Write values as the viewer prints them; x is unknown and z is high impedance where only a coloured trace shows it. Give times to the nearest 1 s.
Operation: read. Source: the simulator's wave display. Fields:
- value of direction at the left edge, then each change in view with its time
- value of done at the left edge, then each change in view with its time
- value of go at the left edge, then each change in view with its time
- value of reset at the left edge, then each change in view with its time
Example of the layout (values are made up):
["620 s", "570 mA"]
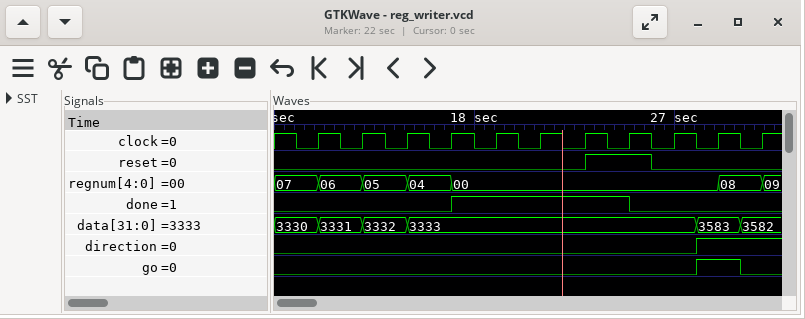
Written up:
["0, 1 at 28 s", "0, 1 at 17 s, 0 at 25 s", "0, 1 at 28 s, 0 at 30 s", "0, 1 at 23 s, 0 at 26 s"]
